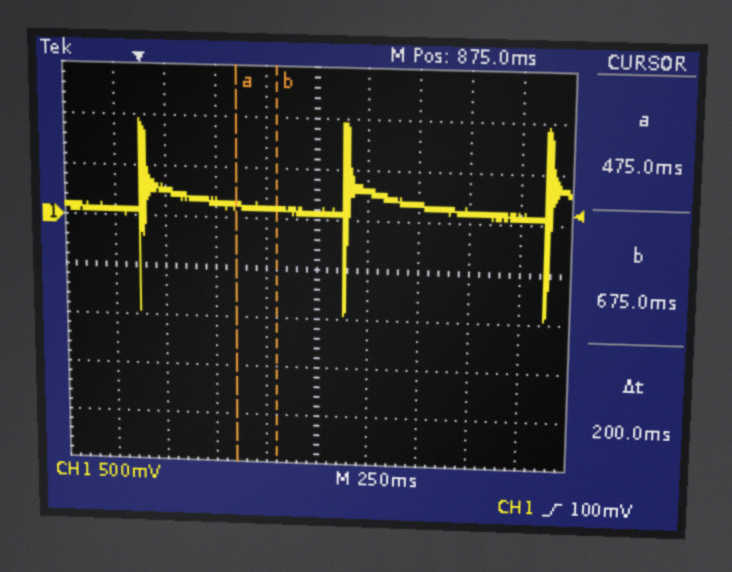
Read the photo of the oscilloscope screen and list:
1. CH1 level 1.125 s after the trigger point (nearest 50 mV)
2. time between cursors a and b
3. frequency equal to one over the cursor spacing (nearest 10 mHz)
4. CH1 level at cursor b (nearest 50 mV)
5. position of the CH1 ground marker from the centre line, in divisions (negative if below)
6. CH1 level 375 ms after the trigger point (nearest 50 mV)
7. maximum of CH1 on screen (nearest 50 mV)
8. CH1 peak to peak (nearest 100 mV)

300 mV
200 ms
5.00 Hz
100 mV
+1.0 div
150 mV
950 mV
1.90 V
